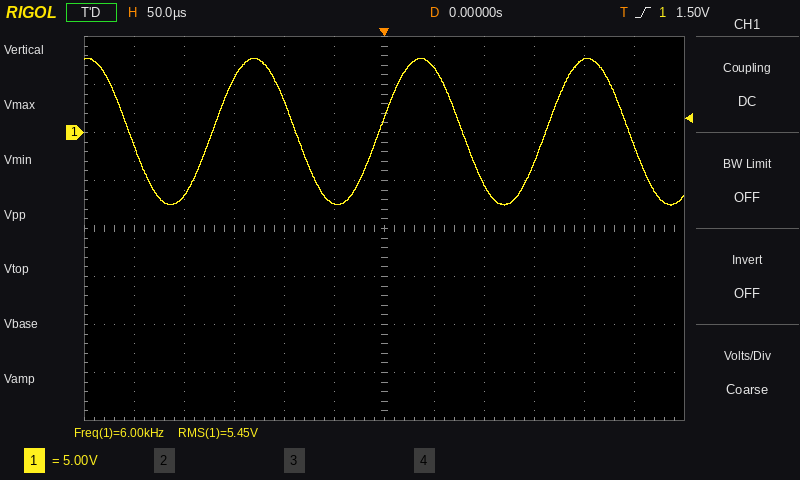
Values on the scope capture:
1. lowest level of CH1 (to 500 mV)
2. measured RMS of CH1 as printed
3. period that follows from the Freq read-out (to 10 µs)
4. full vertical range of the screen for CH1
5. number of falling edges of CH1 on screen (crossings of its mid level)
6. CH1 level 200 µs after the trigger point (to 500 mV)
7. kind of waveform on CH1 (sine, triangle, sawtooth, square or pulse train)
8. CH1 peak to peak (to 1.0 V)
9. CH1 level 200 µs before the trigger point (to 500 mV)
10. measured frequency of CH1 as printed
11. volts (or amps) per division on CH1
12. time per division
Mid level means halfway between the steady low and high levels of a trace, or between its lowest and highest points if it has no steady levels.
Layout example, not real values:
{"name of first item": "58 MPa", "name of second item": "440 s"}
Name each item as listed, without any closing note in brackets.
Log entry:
{"lowest level of CH1": "-7.5 V", "measured RMS of CH1 as printed": "5.45 V", "period that follows from the Freq read-out": "170 µs", "full vertical range of the screen for CH1": "40 V", "number of falling edges of CH1 on screen": "4", "CH1 level 200 µs after the trigger point": "7.5 V", "kind of waveform on CH1": "sine", "CH1 peak to peak": "15.0 V", "CH1 level 200 µs before the trigger point": "-6.5 V", "measured frequency of CH1 as printed": "6.00 kHz", "volts (or amps) per division on CH1": "5 V", "time per division": "50 µs"}
